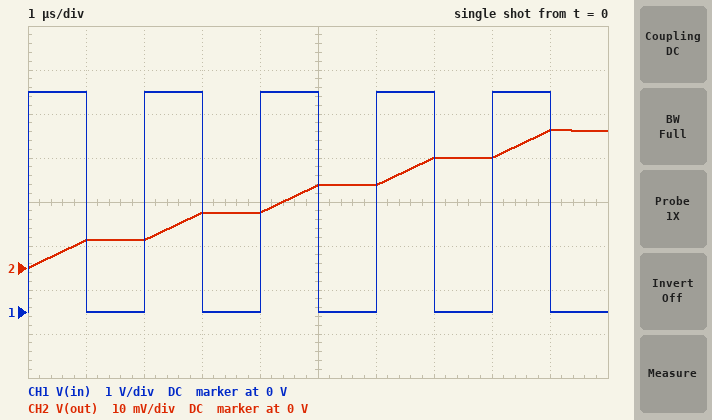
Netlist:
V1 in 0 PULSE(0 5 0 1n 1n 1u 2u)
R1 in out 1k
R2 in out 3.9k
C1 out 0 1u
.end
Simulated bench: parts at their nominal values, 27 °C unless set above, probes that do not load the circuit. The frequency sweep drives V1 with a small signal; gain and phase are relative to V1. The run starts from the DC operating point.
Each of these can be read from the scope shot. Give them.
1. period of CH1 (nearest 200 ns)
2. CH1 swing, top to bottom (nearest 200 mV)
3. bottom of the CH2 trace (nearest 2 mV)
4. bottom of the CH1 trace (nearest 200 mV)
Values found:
2.0 µs
5.0 V
0 V
0 V
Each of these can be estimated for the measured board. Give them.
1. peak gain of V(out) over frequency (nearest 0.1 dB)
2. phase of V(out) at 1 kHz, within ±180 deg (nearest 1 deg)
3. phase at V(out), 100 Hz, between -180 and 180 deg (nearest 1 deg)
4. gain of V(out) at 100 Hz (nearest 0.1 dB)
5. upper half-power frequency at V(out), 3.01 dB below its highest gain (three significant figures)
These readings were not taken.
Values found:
0 dB
-79 deg
-27 deg
-1.0 dB
200 Hz
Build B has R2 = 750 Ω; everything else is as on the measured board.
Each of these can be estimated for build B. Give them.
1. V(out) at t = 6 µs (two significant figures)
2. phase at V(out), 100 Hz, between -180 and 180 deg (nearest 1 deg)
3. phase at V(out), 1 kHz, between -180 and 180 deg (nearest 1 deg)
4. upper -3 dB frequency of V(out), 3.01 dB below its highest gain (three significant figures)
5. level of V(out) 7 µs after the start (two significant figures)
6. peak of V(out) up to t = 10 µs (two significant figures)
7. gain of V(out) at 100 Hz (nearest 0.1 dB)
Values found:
35 mV
-15 deg
-70 deg
371 Hz
46 mV
58 mV
-0.3 dB
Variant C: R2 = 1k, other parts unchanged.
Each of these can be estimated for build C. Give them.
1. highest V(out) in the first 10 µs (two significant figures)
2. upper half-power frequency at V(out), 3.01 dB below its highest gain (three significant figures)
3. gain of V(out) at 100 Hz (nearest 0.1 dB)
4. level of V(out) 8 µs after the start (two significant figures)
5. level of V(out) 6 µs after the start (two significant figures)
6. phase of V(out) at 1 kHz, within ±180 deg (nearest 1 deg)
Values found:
50 mV
318 Hz
-0.4 dB
40 mV
30 mV
-72 deg
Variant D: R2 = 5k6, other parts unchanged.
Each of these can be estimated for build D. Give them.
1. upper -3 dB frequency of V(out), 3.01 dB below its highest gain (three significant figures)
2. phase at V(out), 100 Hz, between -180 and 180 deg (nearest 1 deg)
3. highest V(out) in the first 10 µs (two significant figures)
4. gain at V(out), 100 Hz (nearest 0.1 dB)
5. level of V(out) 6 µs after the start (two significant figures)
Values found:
188 Hz
-28 deg
29 mV
-1.1 dB
18 mV
